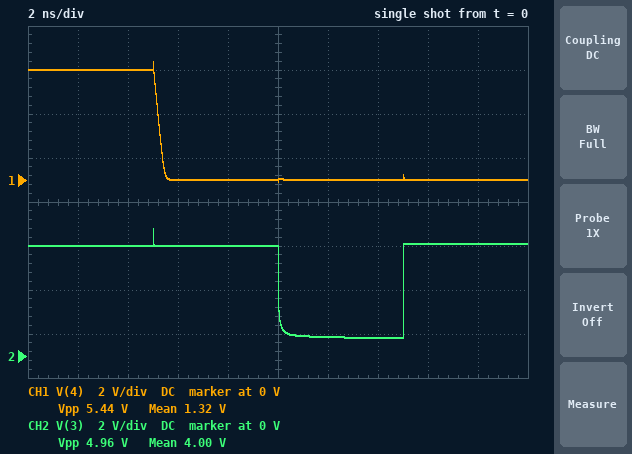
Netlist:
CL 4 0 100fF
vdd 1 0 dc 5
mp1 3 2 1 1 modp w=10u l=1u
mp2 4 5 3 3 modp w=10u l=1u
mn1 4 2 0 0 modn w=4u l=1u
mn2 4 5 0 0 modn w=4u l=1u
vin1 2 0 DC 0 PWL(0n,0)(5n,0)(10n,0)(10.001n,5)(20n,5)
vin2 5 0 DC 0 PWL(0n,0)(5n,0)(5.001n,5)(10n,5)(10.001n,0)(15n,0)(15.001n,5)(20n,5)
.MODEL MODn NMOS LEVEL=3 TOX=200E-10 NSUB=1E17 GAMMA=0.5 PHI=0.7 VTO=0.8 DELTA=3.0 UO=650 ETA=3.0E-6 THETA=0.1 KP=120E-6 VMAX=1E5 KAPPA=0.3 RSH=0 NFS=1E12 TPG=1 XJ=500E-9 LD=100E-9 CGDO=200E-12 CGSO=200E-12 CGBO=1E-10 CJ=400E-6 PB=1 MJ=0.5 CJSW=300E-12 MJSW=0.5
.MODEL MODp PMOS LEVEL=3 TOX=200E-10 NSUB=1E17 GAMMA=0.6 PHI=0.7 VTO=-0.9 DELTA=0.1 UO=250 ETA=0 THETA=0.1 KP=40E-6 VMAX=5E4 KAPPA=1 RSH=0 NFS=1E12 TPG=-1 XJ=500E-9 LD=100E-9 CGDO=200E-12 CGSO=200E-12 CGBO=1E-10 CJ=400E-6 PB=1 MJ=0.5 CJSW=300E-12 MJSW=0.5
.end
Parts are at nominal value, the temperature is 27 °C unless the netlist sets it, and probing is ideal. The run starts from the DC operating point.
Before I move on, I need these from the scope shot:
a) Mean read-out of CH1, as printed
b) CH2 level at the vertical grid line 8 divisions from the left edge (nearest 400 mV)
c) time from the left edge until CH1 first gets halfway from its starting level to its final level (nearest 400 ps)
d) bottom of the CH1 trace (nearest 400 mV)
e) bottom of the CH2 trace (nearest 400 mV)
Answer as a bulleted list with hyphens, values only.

- 1.32 V
- 5.2 V
- 5.2 ns
- 0 V
- 800 mV
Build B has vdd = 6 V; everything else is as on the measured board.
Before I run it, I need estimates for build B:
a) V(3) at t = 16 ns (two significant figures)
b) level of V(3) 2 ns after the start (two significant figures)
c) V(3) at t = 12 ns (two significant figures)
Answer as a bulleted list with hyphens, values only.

- 5.7 V
- 6.0 V
- 1.0 V
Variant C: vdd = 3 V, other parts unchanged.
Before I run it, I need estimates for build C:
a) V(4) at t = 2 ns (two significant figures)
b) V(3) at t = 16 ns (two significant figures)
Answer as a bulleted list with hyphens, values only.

- 3.0 V
- 3.5 V
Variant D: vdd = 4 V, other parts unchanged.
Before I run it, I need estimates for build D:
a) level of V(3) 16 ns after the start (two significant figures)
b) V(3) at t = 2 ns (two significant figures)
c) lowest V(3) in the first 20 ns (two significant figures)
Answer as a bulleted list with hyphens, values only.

- 4.5 V
- 4.0 V
- 800 mV
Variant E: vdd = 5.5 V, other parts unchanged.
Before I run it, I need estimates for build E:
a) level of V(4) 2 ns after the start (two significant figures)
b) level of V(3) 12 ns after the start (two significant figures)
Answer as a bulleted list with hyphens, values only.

- 5.5 V
- 860 mV
